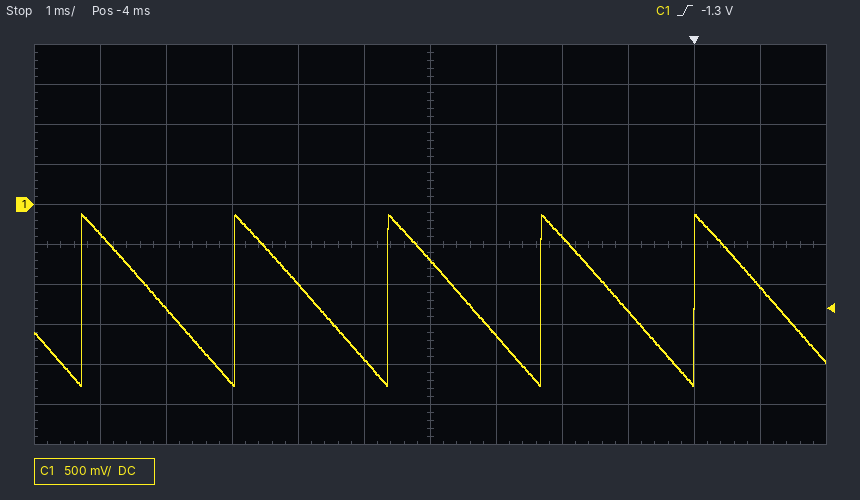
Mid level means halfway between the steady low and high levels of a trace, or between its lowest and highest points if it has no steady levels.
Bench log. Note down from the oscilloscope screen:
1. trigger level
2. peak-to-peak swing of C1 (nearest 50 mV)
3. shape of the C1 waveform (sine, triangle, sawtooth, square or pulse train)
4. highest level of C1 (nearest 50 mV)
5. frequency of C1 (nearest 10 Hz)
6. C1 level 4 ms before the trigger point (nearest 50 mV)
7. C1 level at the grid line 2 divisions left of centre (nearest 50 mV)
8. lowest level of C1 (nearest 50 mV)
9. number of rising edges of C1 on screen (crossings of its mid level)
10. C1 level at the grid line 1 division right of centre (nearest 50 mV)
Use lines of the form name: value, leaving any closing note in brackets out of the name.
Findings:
trigger level: -1.3 V
peak-to-peak swing of C1: 2.15 V
shape of the C1 waveform: sawtooth
highest level of C1: -100 mV
frequency of C1: 430 Hz
C1 level 4 ms before the trigger point: -700 mV
C1 level at the grid line 2 divisions left of centre: -1.00 V
lowest level of C1: -2.25 V
number of rising edges of C1 on screen: 5
C1 level at the grid line 1 division right of centre: -1.65 V
